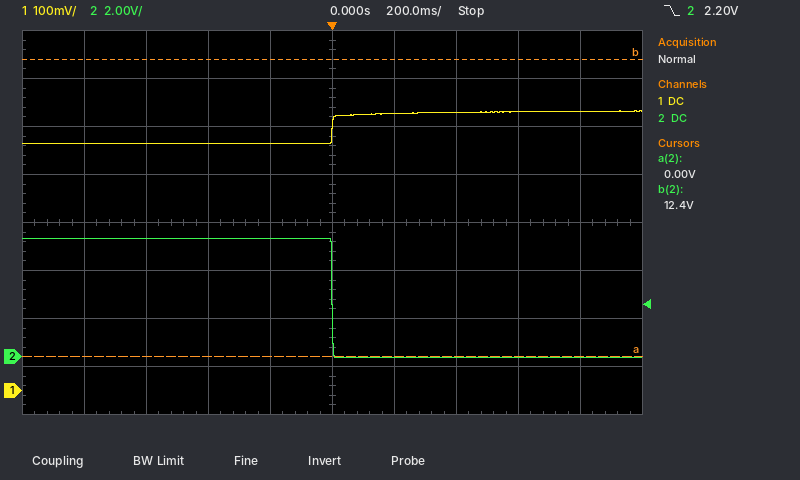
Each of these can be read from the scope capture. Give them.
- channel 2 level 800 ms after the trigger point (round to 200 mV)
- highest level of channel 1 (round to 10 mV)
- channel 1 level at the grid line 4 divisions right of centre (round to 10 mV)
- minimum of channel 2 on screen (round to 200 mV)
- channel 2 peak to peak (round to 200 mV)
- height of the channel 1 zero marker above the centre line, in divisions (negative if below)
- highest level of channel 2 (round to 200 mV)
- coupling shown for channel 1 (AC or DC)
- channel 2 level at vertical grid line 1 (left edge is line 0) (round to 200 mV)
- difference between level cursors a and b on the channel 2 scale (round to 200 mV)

0.0 V
580 mV
580 mV
0.0 V
5.0 V
-3.5 div
5.0 V
DC
5.0 V
12.4 V
